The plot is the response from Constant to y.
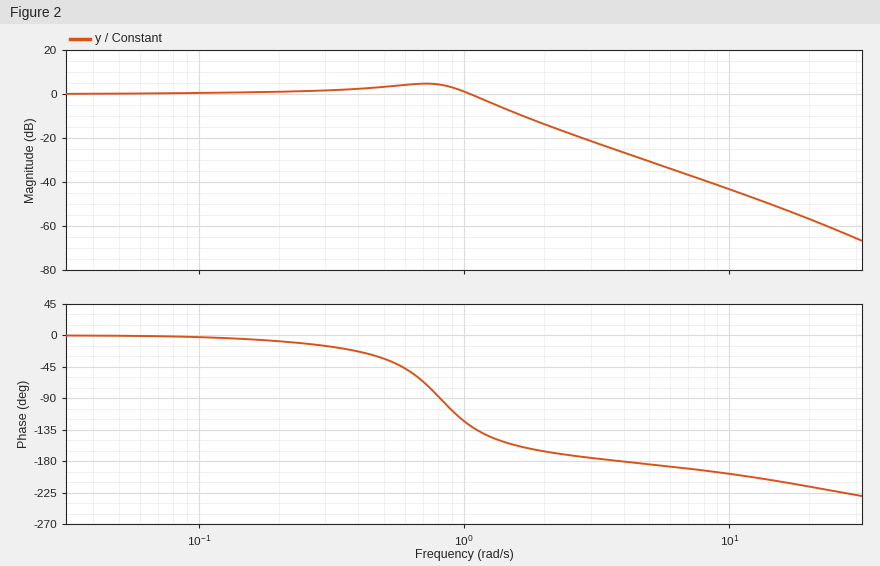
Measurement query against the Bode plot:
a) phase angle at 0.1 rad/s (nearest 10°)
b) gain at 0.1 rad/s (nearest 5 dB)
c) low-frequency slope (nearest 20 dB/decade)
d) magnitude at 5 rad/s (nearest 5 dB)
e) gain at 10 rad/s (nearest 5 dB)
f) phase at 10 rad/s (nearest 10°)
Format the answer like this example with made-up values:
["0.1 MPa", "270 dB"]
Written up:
["0°", "0 dB", "0 dB/decade", "-30 dB", "-45 dB", "-200°"]
